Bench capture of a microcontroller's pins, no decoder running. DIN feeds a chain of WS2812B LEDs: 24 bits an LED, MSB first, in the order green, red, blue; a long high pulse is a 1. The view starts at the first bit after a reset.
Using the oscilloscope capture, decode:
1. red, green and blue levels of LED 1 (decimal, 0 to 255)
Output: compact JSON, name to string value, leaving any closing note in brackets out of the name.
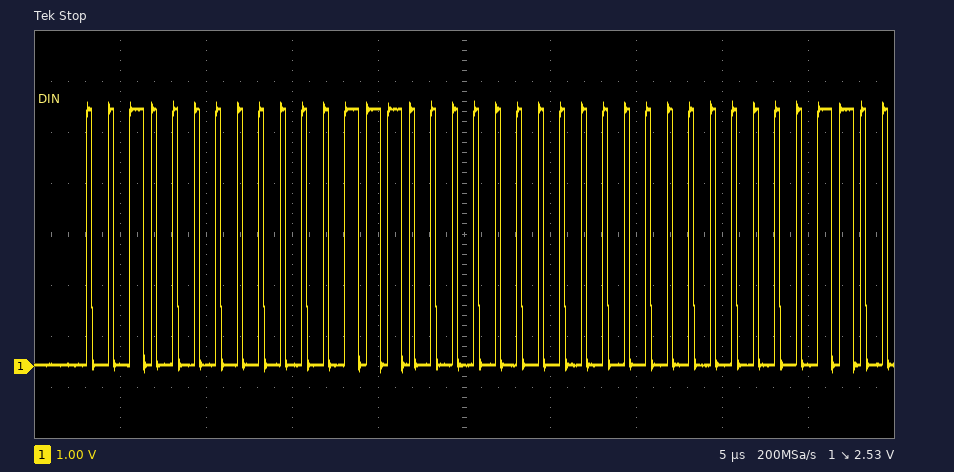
{"red, green and blue levels of LED 1": "14, 32, 0"}
